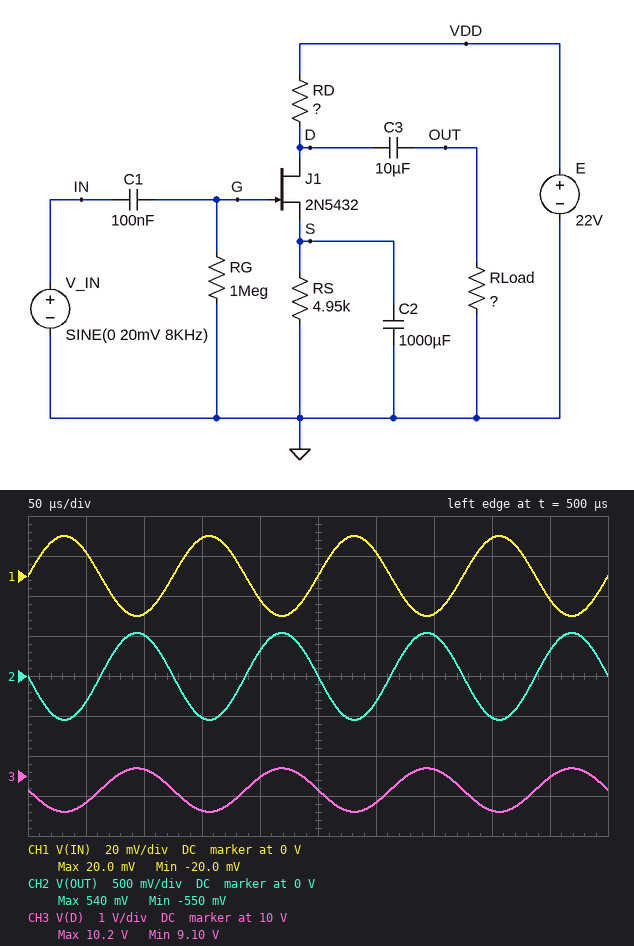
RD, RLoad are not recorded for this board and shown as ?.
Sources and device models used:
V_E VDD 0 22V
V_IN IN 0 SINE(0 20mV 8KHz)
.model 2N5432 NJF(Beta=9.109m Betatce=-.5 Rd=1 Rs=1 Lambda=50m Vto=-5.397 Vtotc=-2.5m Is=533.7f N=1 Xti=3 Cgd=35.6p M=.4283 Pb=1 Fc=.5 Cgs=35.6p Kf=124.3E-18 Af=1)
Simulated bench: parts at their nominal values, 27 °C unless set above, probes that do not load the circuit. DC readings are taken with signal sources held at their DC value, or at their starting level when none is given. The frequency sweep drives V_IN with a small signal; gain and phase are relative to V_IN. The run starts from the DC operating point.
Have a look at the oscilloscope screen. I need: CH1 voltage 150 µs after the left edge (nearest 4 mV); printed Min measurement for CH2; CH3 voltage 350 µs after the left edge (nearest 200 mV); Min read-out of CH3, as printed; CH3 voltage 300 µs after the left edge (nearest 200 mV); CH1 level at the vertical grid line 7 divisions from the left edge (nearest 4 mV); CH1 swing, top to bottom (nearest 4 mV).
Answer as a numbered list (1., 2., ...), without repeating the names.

1. 20 mV
2. -550 mV
3. 10.2 V
4. 9.10 V
5. 9.4 V
6. -20 mV
7. 40 mV
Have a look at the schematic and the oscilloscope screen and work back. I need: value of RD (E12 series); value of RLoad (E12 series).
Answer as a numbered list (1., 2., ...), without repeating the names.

1. 12 kΩ
2. 8.2 kΩ
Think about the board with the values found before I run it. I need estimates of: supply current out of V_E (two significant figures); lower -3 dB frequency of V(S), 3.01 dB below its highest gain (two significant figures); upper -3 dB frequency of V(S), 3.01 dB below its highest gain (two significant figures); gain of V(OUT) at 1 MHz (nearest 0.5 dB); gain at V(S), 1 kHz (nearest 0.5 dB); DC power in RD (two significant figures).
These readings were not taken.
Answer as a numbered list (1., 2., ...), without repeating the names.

1. 1.0 mA
2. 480 mHz
3. 3.3 Hz
4. 28.5 dB
5. -61.0 dB
6. 13 mW
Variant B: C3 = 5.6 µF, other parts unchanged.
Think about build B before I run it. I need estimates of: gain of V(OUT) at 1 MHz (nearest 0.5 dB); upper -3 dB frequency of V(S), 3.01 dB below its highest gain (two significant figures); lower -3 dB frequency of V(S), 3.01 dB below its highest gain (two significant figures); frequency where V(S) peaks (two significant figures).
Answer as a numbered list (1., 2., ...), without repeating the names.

1. 28.5 dB
2. 3.4 Hz
3. 450 mHz
4. 1.2 Hz
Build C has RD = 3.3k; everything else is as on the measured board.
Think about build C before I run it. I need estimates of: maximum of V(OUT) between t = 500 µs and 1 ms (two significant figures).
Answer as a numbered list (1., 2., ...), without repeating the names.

1. 340 mV
